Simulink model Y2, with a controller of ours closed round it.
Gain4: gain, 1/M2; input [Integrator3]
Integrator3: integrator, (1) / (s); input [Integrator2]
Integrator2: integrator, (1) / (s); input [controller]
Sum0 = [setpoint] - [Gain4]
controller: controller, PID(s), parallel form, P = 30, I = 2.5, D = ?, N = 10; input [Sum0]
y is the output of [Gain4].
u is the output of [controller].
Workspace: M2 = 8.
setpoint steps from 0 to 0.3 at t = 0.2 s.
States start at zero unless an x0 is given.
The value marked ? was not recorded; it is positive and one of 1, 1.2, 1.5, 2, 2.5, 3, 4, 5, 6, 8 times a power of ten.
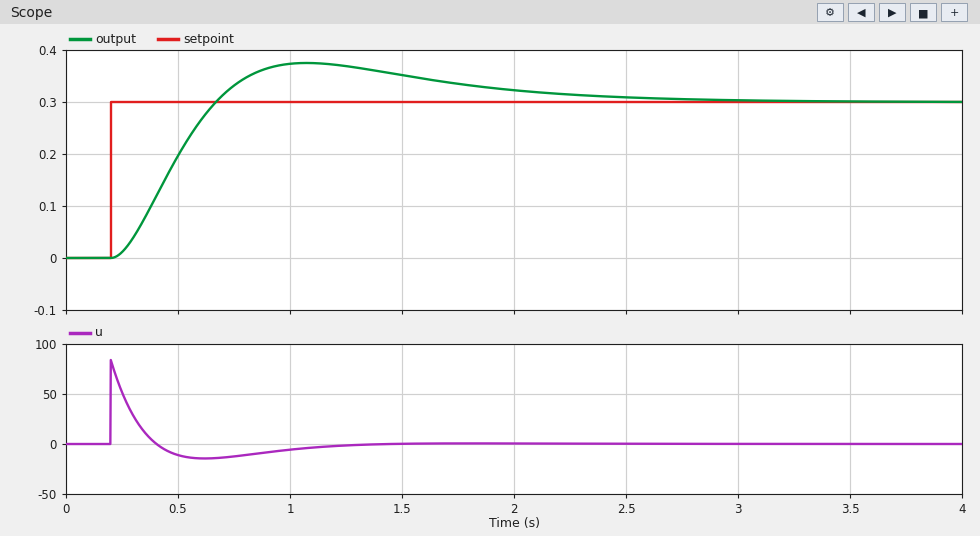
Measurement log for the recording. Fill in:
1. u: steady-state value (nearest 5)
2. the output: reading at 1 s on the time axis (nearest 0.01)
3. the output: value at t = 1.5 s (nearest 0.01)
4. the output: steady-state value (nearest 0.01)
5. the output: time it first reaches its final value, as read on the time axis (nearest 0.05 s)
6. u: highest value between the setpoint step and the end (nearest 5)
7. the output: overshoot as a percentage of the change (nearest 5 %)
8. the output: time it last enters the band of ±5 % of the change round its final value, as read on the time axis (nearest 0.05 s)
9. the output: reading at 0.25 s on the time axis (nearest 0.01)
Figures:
0
0.37
0.35
0.30
0.65 s
85
25 %
2.25 s
0.01
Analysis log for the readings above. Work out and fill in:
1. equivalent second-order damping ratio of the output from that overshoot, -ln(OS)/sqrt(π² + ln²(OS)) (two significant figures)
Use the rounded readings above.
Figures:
0.40
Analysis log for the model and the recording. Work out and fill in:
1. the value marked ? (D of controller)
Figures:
25
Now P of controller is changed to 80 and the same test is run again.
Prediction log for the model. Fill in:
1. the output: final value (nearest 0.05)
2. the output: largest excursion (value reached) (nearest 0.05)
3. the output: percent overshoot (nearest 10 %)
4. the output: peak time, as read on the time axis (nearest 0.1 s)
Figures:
0.30
0.45
40 %
0.9 s
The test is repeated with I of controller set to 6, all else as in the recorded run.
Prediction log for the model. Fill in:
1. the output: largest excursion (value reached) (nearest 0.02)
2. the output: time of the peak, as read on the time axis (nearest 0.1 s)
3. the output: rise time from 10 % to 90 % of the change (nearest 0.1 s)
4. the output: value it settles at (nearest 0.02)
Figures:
0.38
1.1 s
0.3 s
0.30
